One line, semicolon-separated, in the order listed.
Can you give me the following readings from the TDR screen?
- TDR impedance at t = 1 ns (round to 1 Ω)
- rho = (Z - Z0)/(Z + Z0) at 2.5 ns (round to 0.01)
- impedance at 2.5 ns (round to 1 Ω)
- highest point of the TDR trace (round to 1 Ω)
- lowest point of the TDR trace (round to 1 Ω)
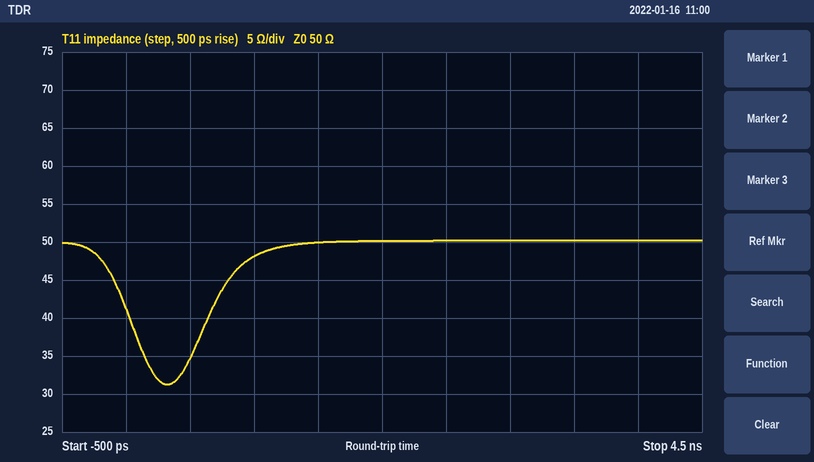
48 Ω; 0.00; 50 Ω; 50 Ω; 31 Ω
